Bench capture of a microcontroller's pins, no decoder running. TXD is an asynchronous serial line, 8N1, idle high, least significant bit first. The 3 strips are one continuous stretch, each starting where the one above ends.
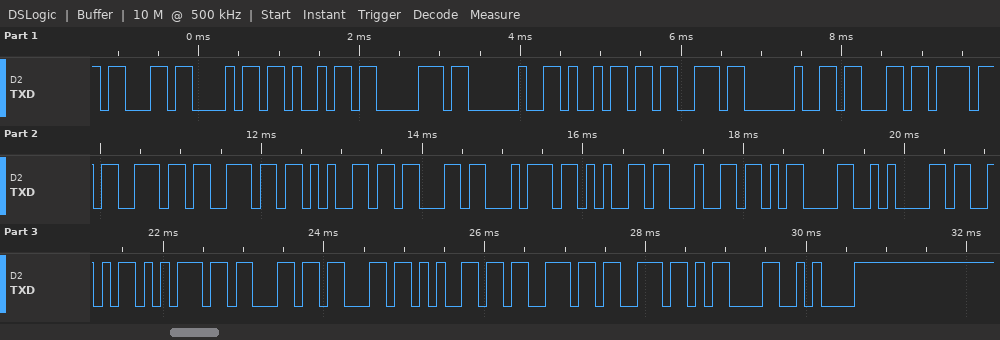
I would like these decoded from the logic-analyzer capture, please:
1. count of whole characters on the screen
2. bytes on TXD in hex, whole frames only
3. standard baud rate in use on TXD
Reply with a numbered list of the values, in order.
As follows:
1. 28
2. 0x63 0x68 0x69 0x70 0x20 0x69 0x73 0x20 0x63 0x6F 0x6E 0x6E 0x65 0x63 0x74 0x65 0x64 0x0D 0x0A 0x53 0x75 0x63 0x63 0x65 0x73 0x73 0x0D 0x0A
3. 9600 baud
